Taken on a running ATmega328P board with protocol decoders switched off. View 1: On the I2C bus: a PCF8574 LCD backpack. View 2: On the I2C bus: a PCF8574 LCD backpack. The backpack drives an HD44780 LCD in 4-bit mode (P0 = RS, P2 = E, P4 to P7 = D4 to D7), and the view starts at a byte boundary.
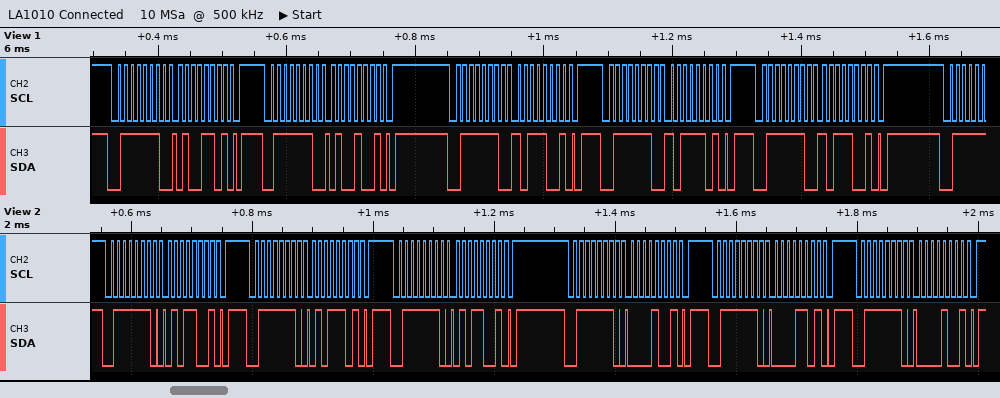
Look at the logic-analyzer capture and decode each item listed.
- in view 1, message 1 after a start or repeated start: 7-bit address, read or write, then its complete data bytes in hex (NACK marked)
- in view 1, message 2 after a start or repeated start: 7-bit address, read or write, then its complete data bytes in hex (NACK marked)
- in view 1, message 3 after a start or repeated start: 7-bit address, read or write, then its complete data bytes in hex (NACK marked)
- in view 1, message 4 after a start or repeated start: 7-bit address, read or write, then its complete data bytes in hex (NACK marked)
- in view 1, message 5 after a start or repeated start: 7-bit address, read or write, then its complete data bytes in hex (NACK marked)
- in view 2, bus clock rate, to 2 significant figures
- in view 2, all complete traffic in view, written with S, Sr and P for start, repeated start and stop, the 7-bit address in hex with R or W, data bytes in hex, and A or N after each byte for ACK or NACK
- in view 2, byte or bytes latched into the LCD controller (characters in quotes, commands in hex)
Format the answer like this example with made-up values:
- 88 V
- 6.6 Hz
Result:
- 0x3F write: 4D
- 0x3F write: 49
- 0x3F write: B9
- 0x3F write: BD
- 0x3F write: B9
- 100 kHz
- S 3FW A 59 A P S 3FW A 5D A P S 3FW A 59 A P S 3FW A 09 A P S 3FW A 0D A P S 3FW A 09 A P
- 'P'
